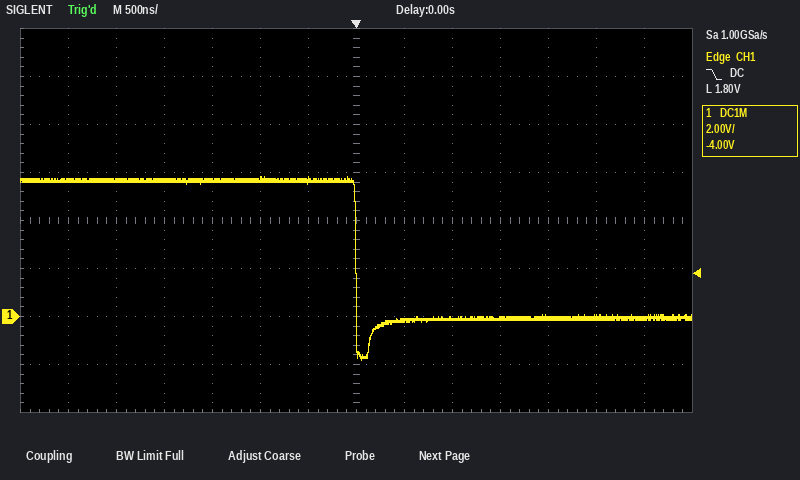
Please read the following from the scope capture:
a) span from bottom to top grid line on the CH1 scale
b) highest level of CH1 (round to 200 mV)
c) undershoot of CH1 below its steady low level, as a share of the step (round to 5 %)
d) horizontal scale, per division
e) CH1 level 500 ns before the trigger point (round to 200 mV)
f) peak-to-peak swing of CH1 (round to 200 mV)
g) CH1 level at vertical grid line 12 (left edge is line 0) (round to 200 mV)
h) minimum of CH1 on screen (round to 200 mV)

16 V
5.8 V
30 %
500 ns
5.6 V
7.6 V
0.0 V
-1.8 V
